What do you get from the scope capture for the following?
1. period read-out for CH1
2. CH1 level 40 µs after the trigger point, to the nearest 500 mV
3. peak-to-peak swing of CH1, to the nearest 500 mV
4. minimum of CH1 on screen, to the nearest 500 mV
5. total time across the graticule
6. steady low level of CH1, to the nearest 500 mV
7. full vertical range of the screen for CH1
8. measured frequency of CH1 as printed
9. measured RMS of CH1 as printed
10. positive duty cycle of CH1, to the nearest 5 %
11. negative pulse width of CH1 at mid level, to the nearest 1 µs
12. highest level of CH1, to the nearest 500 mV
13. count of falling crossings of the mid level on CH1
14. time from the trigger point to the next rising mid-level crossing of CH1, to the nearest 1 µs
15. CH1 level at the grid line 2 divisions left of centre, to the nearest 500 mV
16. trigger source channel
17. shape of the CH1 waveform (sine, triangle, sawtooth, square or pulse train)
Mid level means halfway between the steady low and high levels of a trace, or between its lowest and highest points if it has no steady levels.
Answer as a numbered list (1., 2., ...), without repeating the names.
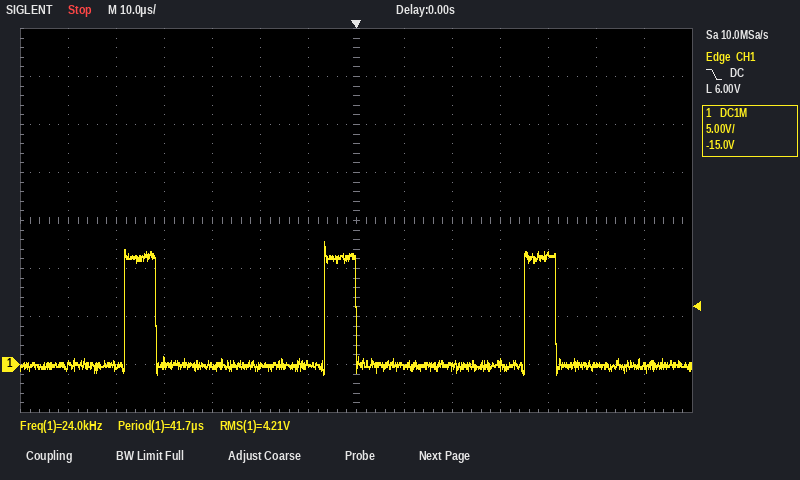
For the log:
1. 41.7 µs
2. 11.5 V
3. 14.0 V
4. -1.0 V
5. 140 µs
6. 0.0 V
7. 40 V
8. 24.0 kHz
9. 4.21 V
10. 15 %
11. 35 µs
12. 13.0 V
13. 3
14. 35 µs
15. 0.0 V
16. CH1
17. pulse train
